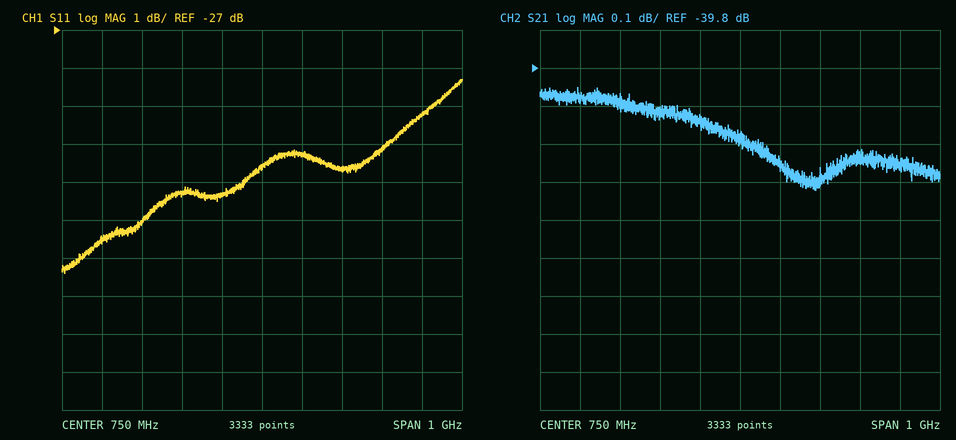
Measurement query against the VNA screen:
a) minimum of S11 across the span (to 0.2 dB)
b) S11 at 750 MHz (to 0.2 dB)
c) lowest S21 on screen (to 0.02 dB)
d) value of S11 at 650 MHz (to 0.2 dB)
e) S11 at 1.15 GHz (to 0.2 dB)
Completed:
-33.4 dB
-30.6 dB
-40.12 dB
-31.4 dB
-29.2 dB
